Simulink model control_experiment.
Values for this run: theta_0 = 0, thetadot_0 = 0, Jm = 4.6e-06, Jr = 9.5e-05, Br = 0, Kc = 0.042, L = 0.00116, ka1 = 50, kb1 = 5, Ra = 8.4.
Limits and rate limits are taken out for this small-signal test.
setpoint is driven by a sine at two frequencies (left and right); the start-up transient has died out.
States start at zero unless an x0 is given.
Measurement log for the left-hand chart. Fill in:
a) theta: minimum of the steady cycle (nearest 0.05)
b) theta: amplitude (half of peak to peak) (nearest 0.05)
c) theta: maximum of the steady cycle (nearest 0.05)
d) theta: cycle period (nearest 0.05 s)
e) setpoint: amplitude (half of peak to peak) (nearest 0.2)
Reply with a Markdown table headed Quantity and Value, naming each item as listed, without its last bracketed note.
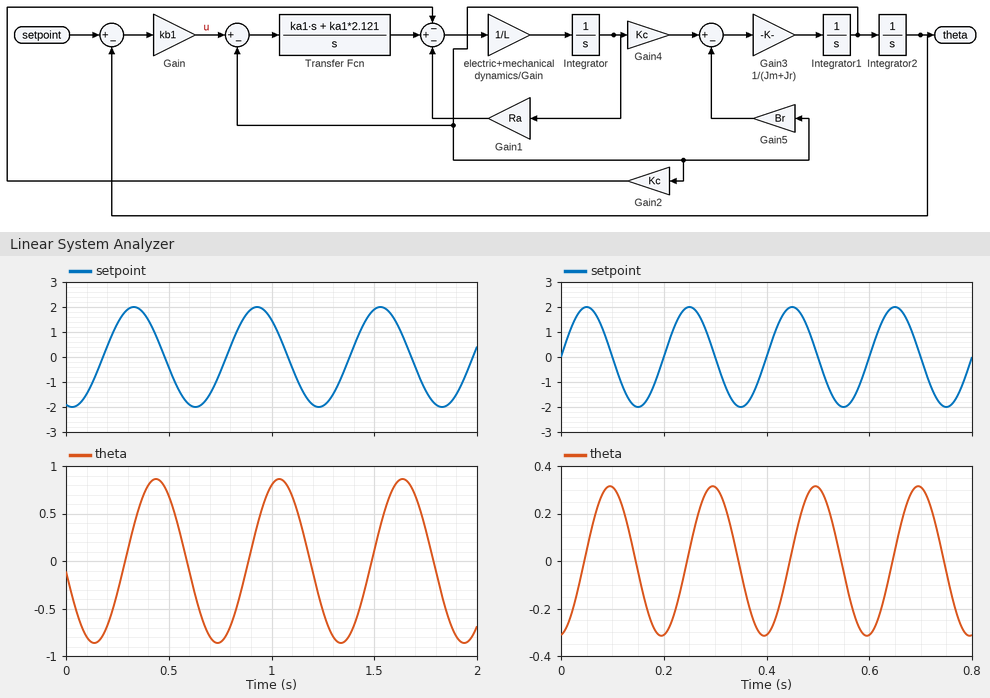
| Quantity | Value |
|---|---|
| theta: minimum of the steady cycle | -0.85 |
| theta: amplitude (half of peak to peak) | 0.85 |
| theta: maximum of the steady cycle | 0.85 |
| theta: cycle period | 0.60 s |
| setpoint: amplitude (half of peak to peak) | 2.0 |
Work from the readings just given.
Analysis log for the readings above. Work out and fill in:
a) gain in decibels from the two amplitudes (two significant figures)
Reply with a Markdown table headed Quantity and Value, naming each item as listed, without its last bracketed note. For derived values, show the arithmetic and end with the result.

| Quantity | Value |
|---|---|
| gain in decibels from the two amplitudes | 20 log10(0.85 / 2) = -7.4 dB |
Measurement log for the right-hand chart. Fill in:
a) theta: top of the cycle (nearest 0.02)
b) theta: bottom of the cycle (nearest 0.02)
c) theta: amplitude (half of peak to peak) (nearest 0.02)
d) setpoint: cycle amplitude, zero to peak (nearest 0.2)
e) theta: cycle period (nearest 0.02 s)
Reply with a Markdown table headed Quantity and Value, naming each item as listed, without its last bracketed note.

| Quantity | Value |
|---|---|
| theta: top of the cycle | 0.32 |
| theta: bottom of the cycle | -0.32 |
| theta: amplitude (half of peak to peak) | 0.32 |
| setpoint: cycle amplitude, zero to peak | 2.0 |
| theta: cycle period | 0.20 s |
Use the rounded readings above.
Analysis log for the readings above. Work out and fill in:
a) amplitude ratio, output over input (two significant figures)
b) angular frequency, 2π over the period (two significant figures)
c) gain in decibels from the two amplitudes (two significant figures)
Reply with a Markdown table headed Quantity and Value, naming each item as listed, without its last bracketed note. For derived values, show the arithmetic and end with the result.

| Quantity | Value |
|---|---|
| amplitude ratio, output over input | 0.32 / 2 = 0.16 |
| angular frequency, 2π over the period | 2π / 0.2 = 31 rad/s |
| gain in decibels from the two amplitudes | 20 log10(0.32 / 2) = -16 dB |
